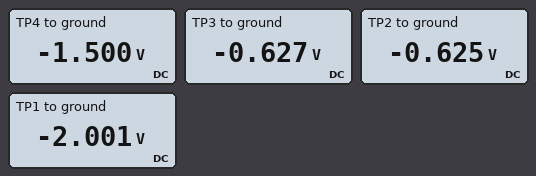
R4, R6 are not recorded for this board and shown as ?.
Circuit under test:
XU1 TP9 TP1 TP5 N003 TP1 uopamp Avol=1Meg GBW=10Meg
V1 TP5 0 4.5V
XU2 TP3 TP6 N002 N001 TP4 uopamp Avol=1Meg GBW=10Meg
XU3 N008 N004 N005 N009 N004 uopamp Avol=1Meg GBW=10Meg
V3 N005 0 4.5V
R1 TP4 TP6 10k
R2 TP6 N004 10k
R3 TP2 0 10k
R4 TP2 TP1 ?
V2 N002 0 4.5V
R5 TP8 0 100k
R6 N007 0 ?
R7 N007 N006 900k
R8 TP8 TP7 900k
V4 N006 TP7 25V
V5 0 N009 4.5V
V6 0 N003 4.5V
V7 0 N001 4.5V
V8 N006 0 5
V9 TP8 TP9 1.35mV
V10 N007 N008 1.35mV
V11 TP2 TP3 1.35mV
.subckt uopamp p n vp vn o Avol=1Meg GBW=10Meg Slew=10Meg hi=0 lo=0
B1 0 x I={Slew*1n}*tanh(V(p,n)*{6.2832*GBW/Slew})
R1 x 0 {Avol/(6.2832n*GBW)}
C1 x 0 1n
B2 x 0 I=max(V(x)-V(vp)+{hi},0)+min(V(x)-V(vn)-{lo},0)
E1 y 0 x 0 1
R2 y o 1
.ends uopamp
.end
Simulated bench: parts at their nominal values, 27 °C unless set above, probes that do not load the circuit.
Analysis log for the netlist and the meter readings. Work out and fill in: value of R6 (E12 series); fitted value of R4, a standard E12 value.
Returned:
47 kΩ
22 kΩ
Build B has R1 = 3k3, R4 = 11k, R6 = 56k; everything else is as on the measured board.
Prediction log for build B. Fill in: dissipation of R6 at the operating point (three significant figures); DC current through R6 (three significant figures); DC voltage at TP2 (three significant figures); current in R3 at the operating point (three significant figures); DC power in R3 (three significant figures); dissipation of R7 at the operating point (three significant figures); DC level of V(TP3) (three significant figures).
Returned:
1.53 µW
5.23 µA
-953 mV
95.3 µA
90.8 µW
24.6 µW
-954 mV
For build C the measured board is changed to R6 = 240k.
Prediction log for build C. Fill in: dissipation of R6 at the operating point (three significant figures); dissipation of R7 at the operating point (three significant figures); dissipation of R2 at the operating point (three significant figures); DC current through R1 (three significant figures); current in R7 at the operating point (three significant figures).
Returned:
4.62 µW
17.3 µW
282 µW
168 µA
4.39 µA
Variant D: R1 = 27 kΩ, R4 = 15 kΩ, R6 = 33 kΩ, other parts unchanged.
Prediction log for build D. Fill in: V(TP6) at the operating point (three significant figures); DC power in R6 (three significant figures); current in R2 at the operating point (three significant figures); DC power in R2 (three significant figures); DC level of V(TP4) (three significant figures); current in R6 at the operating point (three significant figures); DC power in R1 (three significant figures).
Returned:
-802 mV
948 nW
97.7 µA
95.5 µW
-3.44 V
5.36 µA
258 µW
